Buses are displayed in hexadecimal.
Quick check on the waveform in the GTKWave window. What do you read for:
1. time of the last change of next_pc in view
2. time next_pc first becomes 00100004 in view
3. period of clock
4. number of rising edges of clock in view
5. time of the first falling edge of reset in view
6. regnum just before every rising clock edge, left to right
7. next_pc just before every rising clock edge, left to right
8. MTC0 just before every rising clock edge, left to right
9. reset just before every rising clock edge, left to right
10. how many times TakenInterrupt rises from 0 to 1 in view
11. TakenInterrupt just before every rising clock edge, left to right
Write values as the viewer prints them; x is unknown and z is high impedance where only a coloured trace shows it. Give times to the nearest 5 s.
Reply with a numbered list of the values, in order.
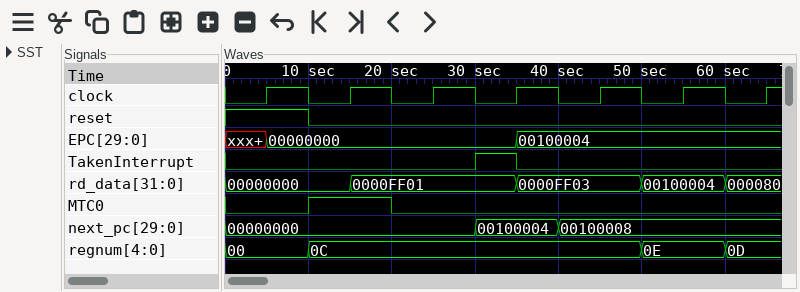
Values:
1. 40 s
2. 30 s
3. 10 s
4. 7
5. 10 s
6. 00, 0C, 0C, 0C, 0C, 0E, 0D
7. 00000000, 00000000, 00000000, 00100004, 00100008, 00100008, 00100008
8. 0 1 0 0 0 0 0
9. 1 0 0 0 0 0 0
10. 1
11. 0 0 0 1 0 0 0
